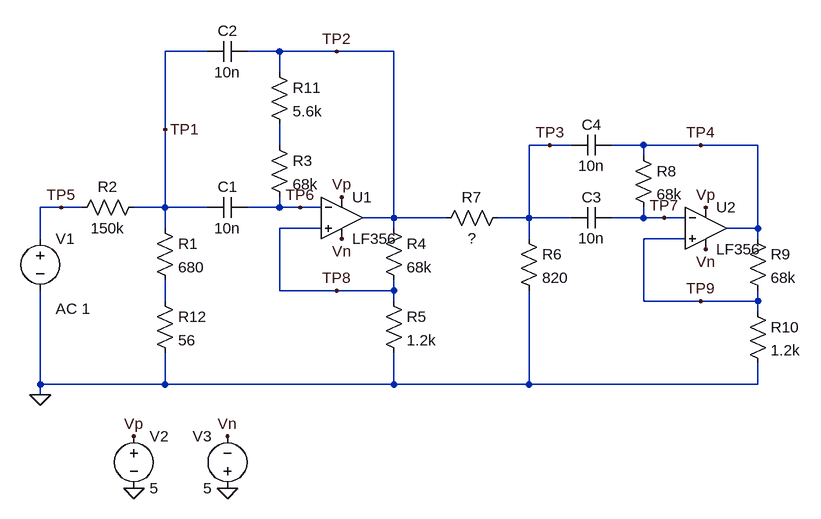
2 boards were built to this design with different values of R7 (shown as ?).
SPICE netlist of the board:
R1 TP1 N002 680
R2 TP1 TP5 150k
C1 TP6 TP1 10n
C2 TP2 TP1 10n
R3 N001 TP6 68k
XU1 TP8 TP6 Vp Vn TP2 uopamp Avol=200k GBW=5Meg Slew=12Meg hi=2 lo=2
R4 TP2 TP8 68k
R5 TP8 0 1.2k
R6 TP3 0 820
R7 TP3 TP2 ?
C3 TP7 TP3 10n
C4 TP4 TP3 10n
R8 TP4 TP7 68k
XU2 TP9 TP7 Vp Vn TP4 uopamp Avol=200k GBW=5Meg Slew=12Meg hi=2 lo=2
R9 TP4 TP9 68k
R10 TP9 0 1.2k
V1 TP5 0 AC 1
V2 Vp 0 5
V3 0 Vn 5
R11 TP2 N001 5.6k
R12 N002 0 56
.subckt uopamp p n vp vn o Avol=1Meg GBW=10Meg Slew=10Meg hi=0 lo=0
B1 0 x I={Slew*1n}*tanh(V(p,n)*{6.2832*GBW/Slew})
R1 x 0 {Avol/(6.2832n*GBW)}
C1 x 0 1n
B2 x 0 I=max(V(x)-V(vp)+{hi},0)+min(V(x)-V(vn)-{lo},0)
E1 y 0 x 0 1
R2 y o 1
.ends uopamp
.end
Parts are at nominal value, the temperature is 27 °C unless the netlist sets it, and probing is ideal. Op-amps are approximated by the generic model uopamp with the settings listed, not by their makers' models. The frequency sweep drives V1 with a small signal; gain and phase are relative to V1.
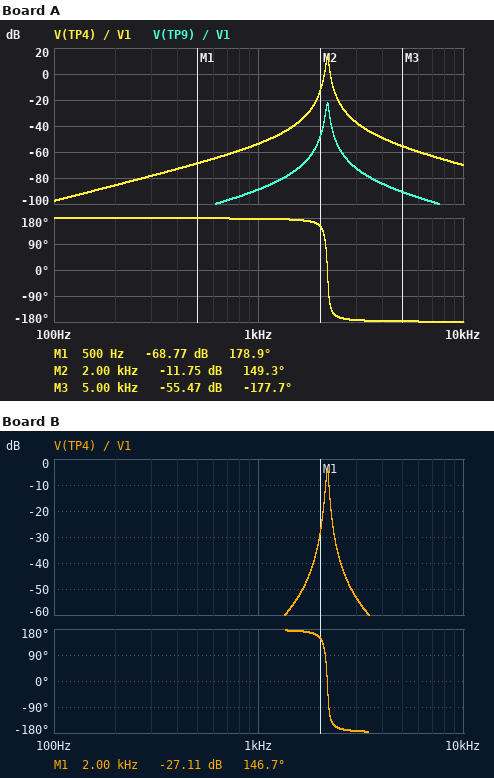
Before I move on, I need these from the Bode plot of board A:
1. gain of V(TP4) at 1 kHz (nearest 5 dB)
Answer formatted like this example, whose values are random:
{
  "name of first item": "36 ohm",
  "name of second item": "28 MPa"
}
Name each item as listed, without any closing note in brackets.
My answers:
{
  "gain of V(TP4) at 1 kHz": "-55 dB"
}
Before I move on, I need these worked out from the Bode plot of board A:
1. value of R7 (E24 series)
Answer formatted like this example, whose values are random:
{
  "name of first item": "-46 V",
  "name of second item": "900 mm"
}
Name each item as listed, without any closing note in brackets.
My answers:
{
  "value of R7": "62 kΩ"
}
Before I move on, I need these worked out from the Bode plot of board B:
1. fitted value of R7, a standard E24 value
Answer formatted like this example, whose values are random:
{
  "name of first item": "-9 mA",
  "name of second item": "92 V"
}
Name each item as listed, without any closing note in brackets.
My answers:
{
  "fitted value of R7, a standard E24 value": "390 kΩ"
}
